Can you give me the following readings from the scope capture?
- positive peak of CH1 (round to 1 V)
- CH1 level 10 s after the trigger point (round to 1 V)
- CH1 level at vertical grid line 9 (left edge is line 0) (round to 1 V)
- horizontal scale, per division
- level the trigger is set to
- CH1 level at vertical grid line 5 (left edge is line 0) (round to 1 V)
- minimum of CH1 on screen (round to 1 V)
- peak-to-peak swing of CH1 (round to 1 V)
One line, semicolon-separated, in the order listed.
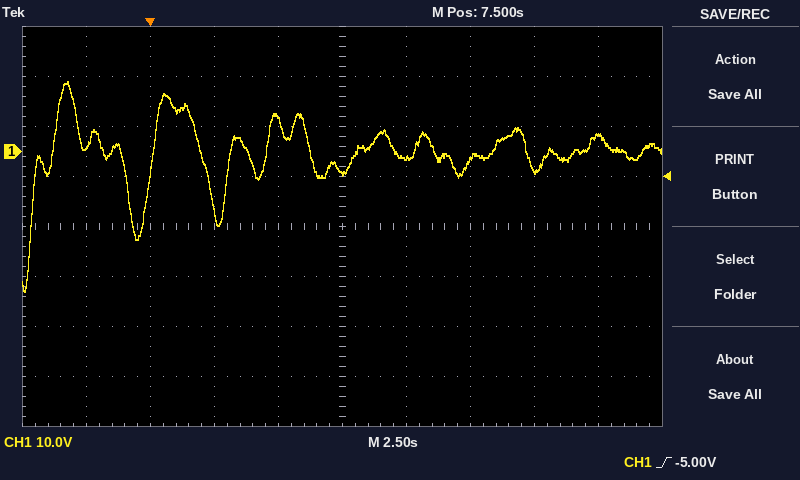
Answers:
14 V; -1 V; 3 V; 2.5 s; -5.00 V; -4 V; -28 V; 42 V
